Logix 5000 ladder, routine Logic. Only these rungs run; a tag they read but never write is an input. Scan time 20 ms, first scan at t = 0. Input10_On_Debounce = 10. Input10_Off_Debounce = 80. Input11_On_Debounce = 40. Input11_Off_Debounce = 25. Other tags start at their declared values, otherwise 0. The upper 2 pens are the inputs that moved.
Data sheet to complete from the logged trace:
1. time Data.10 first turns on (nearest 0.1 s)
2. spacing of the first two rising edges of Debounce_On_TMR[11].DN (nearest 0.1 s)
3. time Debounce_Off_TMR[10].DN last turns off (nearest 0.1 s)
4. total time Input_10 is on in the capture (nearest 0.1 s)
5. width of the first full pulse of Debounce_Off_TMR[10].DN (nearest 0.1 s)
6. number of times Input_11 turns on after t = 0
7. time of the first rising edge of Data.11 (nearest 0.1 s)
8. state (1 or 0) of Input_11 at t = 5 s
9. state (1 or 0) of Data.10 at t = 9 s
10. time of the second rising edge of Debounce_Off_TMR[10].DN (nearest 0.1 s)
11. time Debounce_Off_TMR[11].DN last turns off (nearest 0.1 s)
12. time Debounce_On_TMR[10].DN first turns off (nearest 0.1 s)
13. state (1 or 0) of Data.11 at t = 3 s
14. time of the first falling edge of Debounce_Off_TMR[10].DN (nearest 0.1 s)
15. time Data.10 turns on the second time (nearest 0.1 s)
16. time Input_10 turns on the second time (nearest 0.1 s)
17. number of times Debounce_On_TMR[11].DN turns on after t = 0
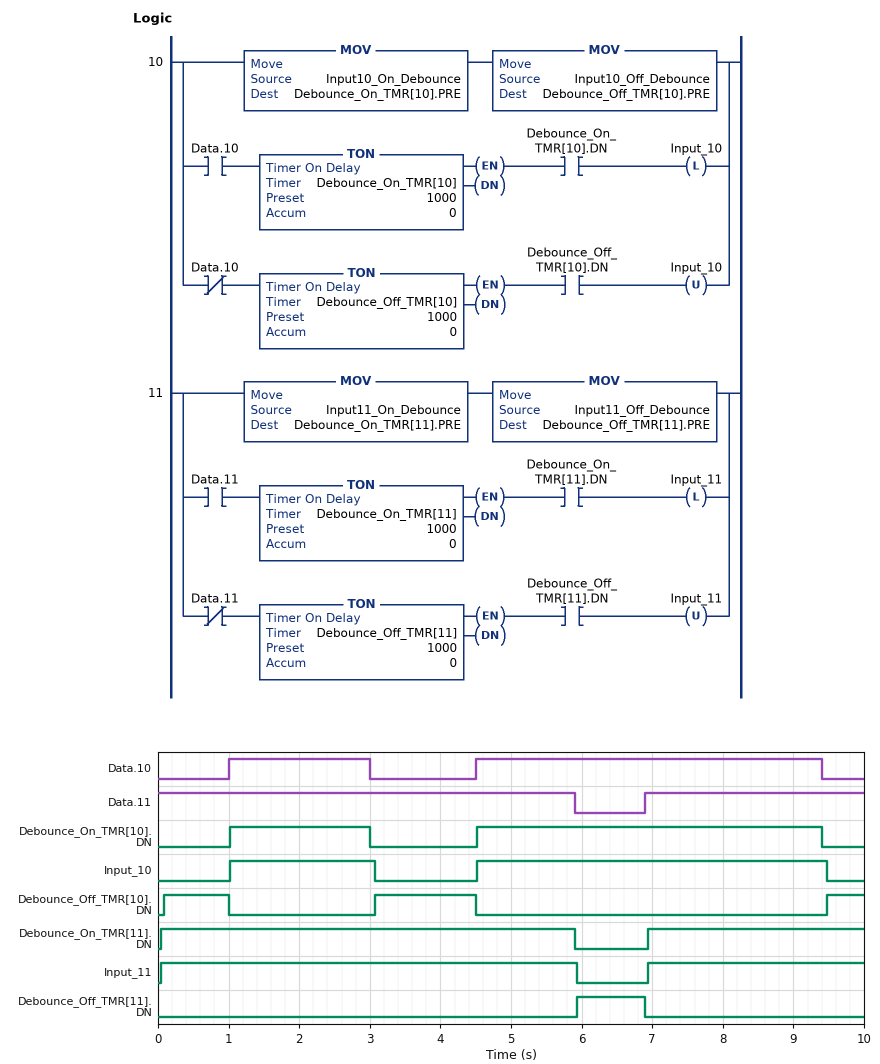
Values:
1.0 s
6.9 s
4.5 s
7.0 s
0.9 s
2
6.9 s
1
1
3.1 s
6.9 s
3.0 s
1
1.0 s
4.5 s
4.5 s
2
